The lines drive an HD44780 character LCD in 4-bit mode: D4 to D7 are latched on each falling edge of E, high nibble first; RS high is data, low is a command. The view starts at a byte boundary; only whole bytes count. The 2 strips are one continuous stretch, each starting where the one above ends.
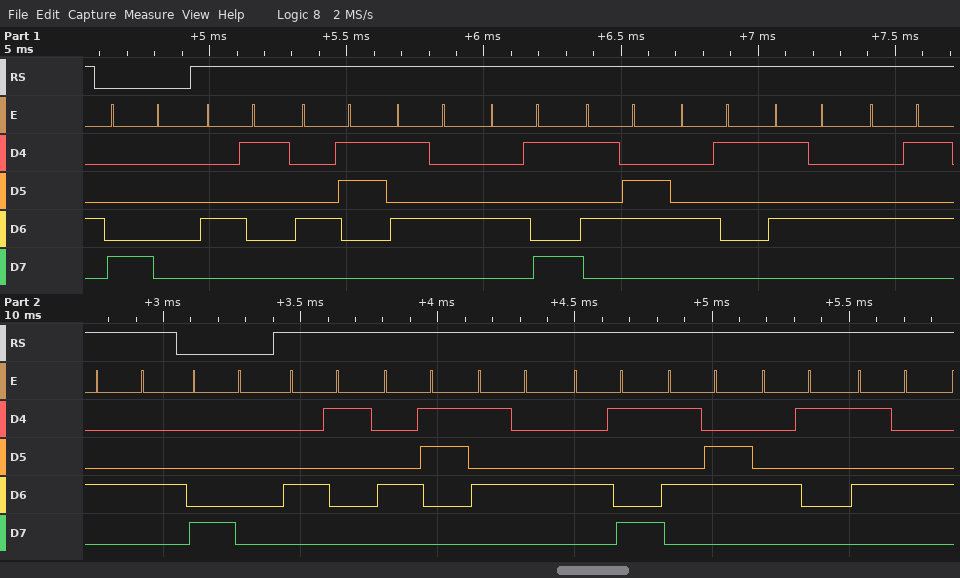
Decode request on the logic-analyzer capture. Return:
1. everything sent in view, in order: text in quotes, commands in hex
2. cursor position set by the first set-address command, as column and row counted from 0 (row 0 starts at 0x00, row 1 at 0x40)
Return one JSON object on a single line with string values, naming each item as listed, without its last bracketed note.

{"everything sent in view, in order: text in quotes, commands in hex": "0x80 \"ACTIVATED\" 0x80 \"ACTIVAT\"", "cursor position set by the first set-address command, as column and row counted from 0": "column 0, row 0"}
